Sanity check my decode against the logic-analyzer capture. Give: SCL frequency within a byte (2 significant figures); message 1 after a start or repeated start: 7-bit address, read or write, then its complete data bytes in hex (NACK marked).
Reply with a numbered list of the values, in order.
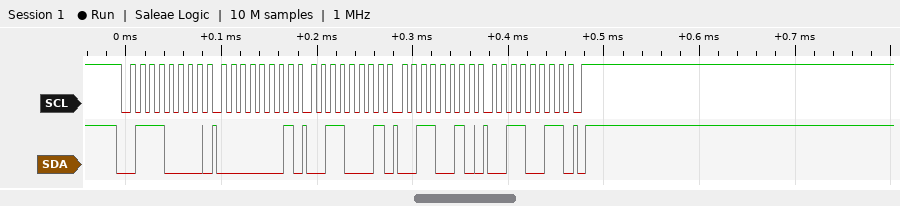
1. 100 kHz
2. 0x38 write: 01 31 32 33
